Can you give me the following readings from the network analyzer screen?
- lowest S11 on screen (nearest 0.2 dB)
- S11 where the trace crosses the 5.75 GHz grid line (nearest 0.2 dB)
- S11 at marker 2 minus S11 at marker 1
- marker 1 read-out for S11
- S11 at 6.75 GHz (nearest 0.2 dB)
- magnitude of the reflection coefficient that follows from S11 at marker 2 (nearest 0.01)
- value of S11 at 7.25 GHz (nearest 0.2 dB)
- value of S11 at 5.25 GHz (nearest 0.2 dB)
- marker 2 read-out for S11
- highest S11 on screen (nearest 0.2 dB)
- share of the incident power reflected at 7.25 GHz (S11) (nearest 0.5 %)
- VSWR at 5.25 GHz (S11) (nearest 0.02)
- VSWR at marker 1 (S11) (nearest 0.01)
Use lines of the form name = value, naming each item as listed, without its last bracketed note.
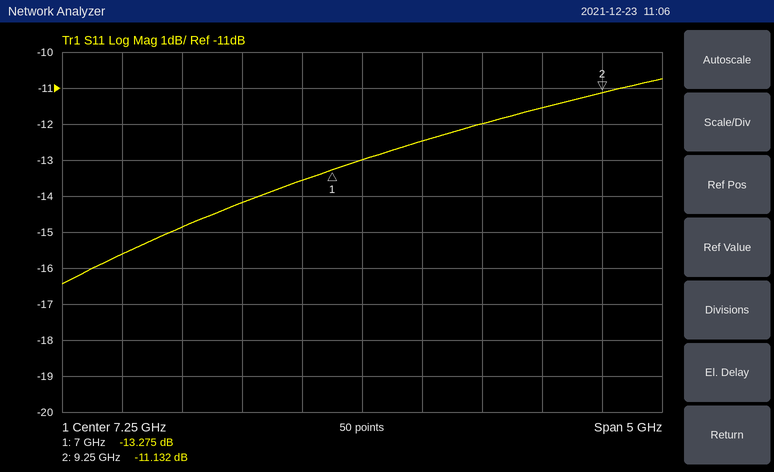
lowest S11 on screen = -16.4 dB
S11 where the trace crosses the 5.75 GHz grid line = -14.8 dB
S11 at marker 2 minus S11 at marker 1 = 2.143 dB
marker 1 read-out for S11 = -13.275 dB
S11 at 6.75 GHz = -13.6 dB
magnitude of the reflection coefficient that follows from S11 at marker 2 = 0.28
value of S11 at 7.25 GHz = -13.0 dB
value of S11 at 5.25 GHz = -15.6 dB
marker 2 read-out for S11 = -11.132 dB
highest S11 on screen = -10.8 dB
share of the incident power reflected at 7.25 GHz (S11) = 5.0 %
VSWR at 5.25 GHz (S11) = 1.40
VSWR at marker 1 (S11) = 1.55
